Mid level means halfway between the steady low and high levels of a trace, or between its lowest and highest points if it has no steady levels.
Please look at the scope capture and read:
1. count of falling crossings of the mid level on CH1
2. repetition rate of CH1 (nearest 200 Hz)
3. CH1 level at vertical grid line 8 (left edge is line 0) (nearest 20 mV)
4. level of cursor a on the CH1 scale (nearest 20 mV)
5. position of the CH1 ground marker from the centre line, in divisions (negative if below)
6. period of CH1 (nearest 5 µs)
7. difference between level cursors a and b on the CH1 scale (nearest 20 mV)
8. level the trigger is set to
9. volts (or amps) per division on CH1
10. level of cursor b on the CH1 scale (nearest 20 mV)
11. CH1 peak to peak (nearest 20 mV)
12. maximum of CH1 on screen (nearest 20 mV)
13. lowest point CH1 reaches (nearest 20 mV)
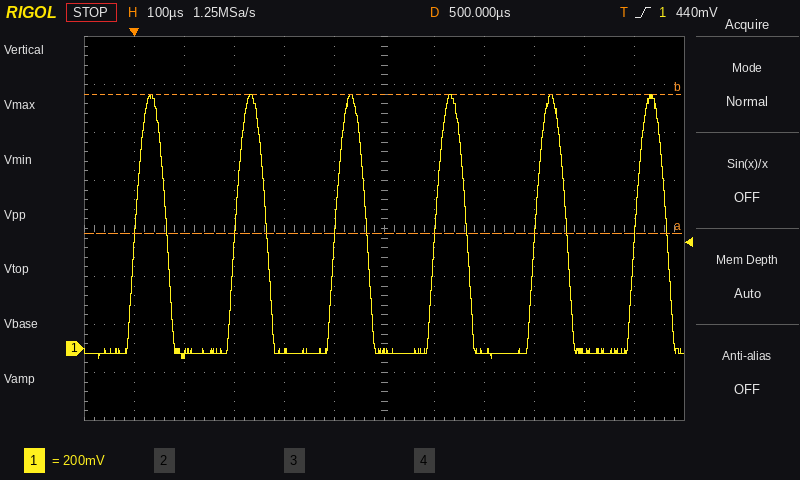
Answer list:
6
5.0 kHz
-20 mV
480 mV
-2.5 div
200 µs
580 mV
440 mV
200 mV
1.06 V
1.10 V
1.06 V
-40 mV
